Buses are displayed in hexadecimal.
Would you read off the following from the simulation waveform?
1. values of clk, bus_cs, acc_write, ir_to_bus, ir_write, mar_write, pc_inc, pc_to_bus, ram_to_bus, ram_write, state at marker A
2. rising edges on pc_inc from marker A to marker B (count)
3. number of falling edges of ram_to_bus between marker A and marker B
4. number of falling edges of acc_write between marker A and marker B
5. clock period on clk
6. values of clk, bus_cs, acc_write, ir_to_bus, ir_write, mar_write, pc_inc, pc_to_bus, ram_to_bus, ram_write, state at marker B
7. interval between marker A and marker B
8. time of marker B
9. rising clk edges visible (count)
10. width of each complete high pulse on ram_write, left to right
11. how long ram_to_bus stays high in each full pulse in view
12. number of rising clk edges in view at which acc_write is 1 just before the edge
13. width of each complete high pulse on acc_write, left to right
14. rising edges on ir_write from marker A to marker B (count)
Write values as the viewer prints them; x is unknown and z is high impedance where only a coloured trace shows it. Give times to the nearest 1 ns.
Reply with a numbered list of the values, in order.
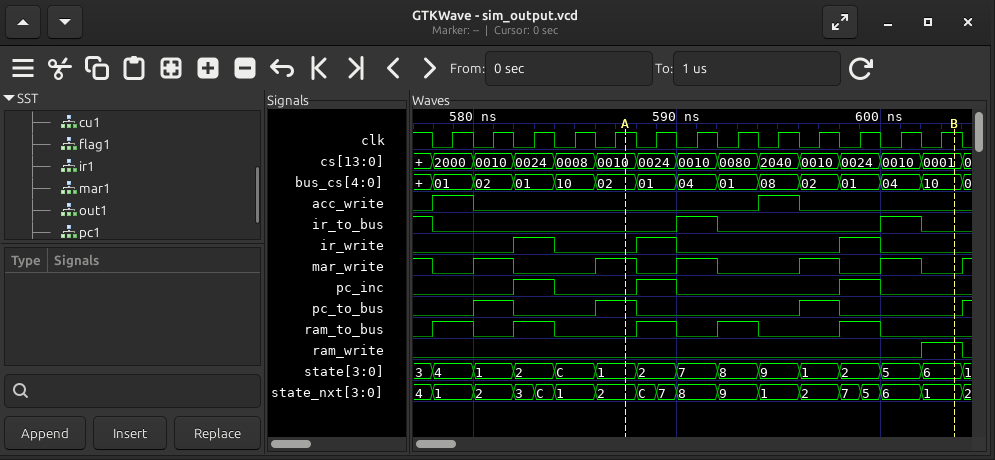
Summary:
1. clk=1, bus_cs=02, acc_write=0, ir_to_bus=0, ir_write=0, mar_write=1, pc_inc=0, pc_to_bus=1, ram_to_bus=0, ram_write=0, state=1
2. 2
3. 3
4. 1
5. 2 ns
6. clk=1, bus_cs=10, acc_write=0, ir_to_bus=0, ir_write=0, mar_write=0, pc_inc=0, pc_to_bus=0, ram_to_bus=0, ram_write=1, state=6
7. 16 ns
8. 604 ns
9. 13
10. 2 ns
11. 2 ns, 2 ns, 2 ns, 2 ns, 2 ns
12. 2
13. 2 ns, 2 ns
14. 2
